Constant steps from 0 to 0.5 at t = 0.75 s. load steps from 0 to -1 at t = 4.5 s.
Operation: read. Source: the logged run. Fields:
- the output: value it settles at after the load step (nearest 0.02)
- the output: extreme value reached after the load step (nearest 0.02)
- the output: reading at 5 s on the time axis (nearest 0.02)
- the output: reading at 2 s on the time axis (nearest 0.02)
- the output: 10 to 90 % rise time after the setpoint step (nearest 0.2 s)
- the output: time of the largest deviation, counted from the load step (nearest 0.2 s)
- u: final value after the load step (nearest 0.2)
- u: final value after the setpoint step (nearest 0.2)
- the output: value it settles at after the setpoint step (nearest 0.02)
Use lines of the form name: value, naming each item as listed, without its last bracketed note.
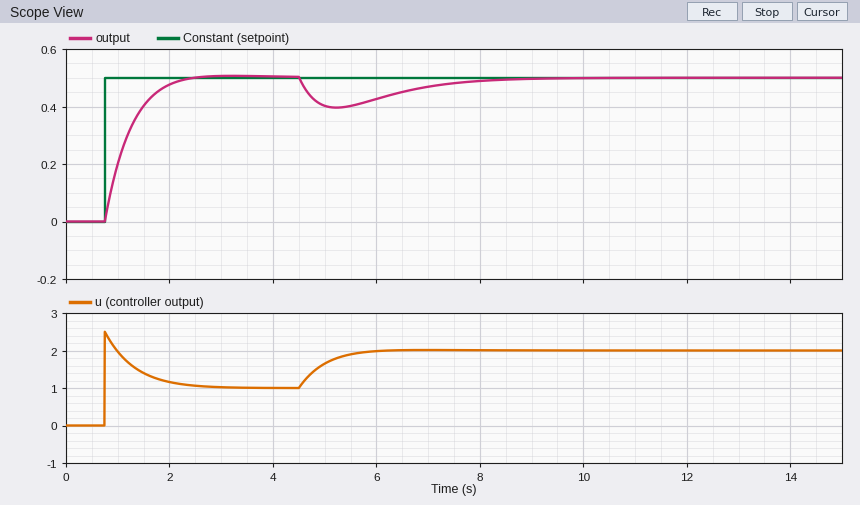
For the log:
the output: value it settles at after the load step: 0.50
the output: extreme value reached after the load step: 0.40
the output: reading at 5 s on the time axis: 0.40
the output: reading at 2 s on the time axis: 0.48
the output: 10 to 90 % rise time after the setpoint step: 1.0 s
the output: time of the largest deviation, counted from the load step: 0.8 s
u: final value after the load step: 2.0
u: final value after the setpoint step: 1.0
the output: value it settles at after the setpoint step: 0.50
